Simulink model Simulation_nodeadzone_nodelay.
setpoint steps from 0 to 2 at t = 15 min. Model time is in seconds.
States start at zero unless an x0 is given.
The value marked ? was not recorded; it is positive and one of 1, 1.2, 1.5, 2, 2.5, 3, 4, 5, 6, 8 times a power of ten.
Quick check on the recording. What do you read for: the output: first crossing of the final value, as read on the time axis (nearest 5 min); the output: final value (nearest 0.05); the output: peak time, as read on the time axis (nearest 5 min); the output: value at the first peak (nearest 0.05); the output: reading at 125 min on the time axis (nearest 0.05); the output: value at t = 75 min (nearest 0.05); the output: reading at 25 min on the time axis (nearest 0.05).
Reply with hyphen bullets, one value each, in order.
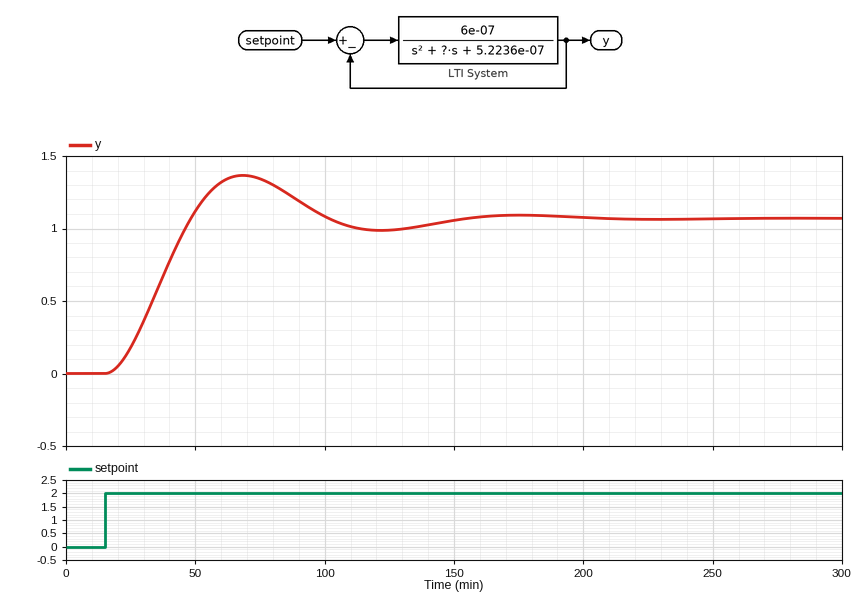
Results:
- 50 min
- 1.05
- 70 min
- 1.35
- 1.00
- 1.35
- 0.20
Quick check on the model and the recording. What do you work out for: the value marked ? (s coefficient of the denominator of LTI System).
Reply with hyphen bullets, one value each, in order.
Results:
- 0.0008
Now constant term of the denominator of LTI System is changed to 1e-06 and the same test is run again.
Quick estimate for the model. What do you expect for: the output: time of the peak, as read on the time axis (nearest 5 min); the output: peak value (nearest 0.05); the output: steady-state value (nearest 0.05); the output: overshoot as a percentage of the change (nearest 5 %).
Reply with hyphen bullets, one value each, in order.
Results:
- 60 min
- 1.00
- 0.75
- 35 %
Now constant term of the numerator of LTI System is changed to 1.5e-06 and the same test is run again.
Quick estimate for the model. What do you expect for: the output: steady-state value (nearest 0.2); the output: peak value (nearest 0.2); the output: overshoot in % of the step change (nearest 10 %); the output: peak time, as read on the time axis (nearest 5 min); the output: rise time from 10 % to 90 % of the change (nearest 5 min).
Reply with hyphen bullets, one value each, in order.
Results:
- 1.4
- 2.0
- 40 %
- 55 min
- 15 min
